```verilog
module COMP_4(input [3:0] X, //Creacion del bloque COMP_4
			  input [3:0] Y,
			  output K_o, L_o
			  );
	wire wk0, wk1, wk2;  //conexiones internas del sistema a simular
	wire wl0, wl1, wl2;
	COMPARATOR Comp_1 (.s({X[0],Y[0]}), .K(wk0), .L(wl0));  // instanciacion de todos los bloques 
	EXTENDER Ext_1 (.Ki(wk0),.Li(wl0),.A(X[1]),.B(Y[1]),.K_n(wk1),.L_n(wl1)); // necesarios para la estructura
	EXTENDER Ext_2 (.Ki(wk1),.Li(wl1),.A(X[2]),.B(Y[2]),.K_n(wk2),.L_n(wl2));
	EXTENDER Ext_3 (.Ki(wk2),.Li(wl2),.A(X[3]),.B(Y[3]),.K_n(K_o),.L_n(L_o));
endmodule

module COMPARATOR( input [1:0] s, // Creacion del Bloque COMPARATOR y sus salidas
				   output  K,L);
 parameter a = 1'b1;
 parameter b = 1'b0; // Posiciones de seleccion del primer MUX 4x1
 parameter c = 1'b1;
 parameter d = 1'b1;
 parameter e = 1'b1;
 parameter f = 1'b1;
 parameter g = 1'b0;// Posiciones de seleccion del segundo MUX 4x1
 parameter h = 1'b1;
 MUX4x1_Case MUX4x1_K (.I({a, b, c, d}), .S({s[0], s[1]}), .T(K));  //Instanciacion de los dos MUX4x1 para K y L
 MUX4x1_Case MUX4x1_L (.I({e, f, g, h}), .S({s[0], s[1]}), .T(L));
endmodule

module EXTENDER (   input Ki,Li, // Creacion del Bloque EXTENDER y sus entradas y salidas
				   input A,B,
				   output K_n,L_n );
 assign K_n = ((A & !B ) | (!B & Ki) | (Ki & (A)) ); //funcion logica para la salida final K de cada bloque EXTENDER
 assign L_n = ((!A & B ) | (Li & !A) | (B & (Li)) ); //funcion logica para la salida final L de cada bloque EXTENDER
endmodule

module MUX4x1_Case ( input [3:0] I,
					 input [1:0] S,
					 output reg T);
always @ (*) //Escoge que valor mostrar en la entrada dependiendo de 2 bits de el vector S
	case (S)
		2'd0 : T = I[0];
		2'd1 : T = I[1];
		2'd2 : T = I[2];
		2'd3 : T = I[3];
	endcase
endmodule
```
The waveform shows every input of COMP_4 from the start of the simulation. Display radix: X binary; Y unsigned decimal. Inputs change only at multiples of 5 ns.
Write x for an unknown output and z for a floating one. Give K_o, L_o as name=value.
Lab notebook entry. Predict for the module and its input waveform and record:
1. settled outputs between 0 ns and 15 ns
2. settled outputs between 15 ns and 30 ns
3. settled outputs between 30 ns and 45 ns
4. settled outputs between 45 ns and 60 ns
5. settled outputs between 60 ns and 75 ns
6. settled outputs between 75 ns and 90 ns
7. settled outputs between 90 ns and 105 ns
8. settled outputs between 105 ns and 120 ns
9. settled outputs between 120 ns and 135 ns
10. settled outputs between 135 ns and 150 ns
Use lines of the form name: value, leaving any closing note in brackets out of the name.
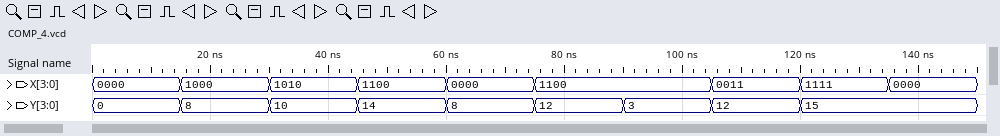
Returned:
settled outputs between 0 ns and 15 ns: K_o=1, L_o=1
settled outputs between 15 ns and 30 ns: K_o=1, L_o=1
settled outputs between 30 ns and 45 ns: K_o=1, L_o=1
settled outputs between 45 ns and 60 ns: K_o=0, L_o=1
settled outputs between 60 ns and 75 ns: K_o=0, L_o=1
settled outputs between 75 ns and 90 ns: K_o=1, L_o=1
settled outputs between 90 ns and 105 ns: K_o=1, L_o=0
settled outputs between 105 ns and 120 ns: K_o=0, L_o=1
settled outputs between 120 ns and 135 ns: K_o=1, L_o=1
settled outputs between 135 ns and 150 ns: K_o=0, L_o=1
